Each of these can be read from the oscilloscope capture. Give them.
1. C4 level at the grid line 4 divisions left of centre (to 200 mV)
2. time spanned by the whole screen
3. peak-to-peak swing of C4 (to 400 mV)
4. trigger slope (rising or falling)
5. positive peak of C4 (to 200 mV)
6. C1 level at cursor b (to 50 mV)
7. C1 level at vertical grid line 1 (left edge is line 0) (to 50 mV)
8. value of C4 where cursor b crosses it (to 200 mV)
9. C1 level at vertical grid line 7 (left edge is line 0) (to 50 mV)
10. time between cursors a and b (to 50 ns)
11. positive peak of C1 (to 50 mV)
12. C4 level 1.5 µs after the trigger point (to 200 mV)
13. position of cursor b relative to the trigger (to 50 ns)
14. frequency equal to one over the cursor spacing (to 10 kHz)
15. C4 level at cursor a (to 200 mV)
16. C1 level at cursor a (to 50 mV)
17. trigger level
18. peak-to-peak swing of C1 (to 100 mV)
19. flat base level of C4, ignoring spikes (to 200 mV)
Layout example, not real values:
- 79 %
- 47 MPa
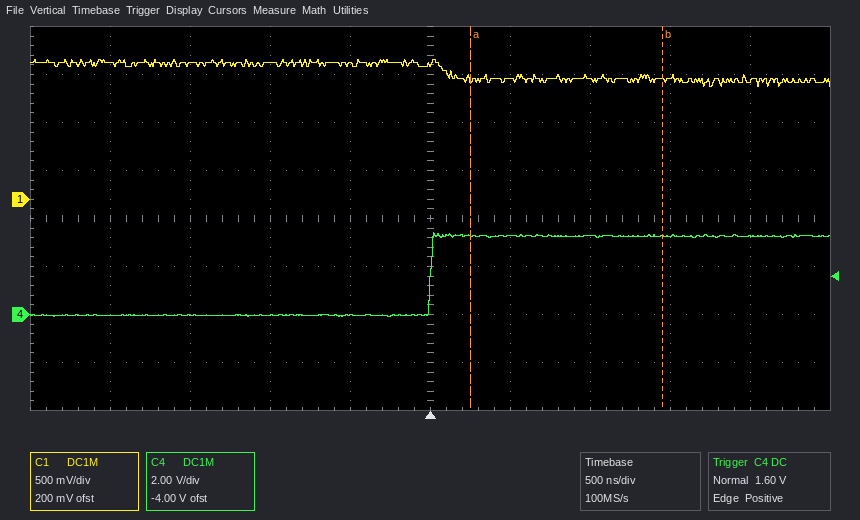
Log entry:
- 0.0 V
- 5 µs
- 3.6 V
- rising
- 3.4 V
- 1.25 V
- 1.40 V
- 3.2 V
- 1.25 V
- 1.20 µs
- 1.45 V
- 3.2 V
- +1.45 µs
- 830 kHz
- 3.2 V
- 1.25 V
- 1.60 V
- 300 mV
- 0.0 V
